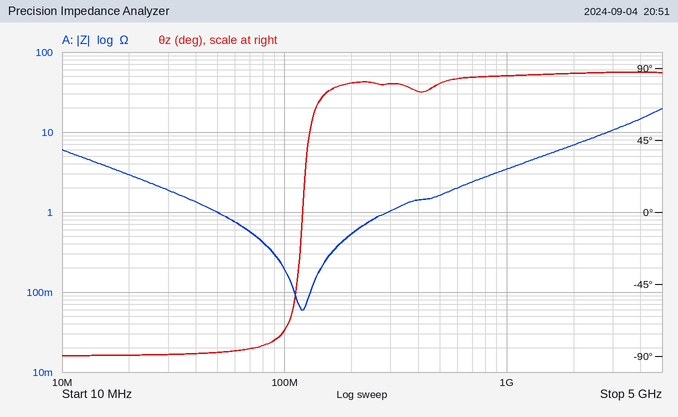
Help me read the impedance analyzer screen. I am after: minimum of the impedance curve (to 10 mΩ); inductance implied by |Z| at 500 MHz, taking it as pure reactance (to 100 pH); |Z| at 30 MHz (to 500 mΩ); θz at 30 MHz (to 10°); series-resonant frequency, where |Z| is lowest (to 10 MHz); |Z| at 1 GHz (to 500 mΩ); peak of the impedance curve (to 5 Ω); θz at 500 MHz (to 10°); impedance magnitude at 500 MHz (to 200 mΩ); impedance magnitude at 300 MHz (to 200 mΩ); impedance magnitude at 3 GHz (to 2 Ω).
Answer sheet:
60 mΩ
500 pH
2.0 Ω
-90°
120 MHz
3.5 Ω
20 Ω
80°
1.6 Ω
1.0 Ω
10 Ω
